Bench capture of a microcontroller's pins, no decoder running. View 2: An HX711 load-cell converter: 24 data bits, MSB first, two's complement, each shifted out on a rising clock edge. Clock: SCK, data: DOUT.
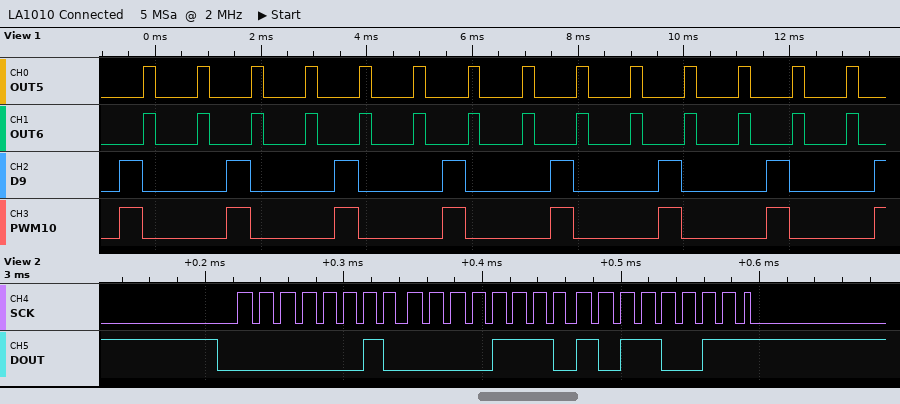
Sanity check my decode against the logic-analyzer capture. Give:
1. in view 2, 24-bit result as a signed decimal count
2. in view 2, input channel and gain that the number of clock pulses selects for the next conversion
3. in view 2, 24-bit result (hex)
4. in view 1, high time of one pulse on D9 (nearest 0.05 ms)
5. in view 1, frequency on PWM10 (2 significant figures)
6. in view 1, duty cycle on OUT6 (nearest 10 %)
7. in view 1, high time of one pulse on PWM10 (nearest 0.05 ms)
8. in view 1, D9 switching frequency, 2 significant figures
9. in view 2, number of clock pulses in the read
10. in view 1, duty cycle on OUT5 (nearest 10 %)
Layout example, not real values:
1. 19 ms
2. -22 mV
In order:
1. 134835
2. channel A, gain 128
3. 0x020EB3
4. 0.45 ms
5. 490 Hz
6. 20 %
7. 0.45 ms
8. 490 Hz
9. 25
10. 20 %
